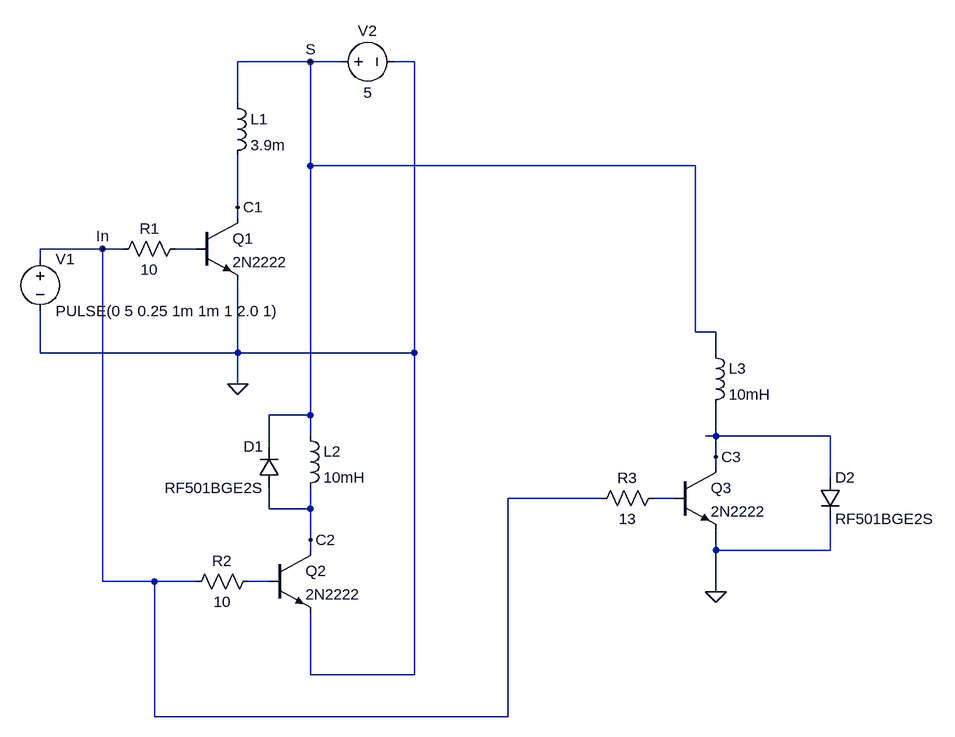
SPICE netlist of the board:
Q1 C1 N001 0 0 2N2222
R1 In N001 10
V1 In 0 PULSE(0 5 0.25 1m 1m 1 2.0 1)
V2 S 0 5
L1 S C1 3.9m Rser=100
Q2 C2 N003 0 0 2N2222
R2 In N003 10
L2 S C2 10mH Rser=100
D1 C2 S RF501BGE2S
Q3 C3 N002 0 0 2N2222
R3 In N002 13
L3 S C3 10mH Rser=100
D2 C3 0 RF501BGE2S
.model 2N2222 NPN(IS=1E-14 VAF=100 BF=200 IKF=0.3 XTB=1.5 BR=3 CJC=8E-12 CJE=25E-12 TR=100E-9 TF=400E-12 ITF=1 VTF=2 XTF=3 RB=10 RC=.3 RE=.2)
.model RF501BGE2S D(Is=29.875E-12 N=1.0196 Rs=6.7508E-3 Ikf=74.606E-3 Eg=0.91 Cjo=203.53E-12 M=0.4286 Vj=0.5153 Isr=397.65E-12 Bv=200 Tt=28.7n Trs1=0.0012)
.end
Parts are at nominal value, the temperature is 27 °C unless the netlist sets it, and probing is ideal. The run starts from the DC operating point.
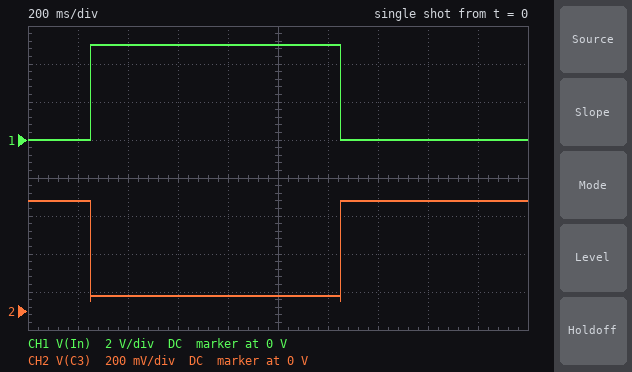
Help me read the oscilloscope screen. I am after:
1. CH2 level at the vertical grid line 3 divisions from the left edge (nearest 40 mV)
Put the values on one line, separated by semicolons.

80 mV
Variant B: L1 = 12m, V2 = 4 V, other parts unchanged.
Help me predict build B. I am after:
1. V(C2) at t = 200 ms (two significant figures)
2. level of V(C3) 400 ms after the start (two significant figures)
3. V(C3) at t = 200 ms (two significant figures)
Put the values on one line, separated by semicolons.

4.0 V; 73 mV; 570 mV
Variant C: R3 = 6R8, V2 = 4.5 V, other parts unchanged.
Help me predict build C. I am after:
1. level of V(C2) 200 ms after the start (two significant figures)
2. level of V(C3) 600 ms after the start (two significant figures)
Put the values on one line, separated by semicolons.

4.5 V; 90 mV
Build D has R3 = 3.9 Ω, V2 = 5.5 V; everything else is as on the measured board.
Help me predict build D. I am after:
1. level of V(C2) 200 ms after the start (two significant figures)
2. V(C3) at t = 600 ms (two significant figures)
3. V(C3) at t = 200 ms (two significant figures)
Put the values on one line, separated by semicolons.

5.5 V; 110 mV; 580 mV
